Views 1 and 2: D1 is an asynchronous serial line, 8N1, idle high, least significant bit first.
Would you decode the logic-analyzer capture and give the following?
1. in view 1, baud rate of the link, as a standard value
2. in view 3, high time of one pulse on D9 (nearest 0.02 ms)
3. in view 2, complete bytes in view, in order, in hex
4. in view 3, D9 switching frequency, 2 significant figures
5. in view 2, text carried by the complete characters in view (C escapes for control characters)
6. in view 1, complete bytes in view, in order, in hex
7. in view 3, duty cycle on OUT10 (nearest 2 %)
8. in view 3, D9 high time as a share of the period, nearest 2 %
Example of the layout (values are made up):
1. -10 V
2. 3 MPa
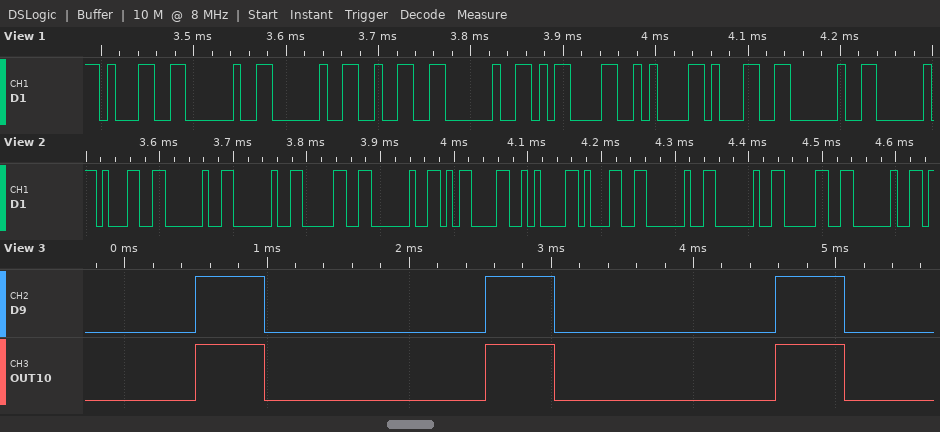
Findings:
1. 115200 baud
2. 0.48 ms
3. 31 20 20 30 20 0D 0A 31 20 20 30 20
4. 490 Hz
5. "1  0 \r\n1  0 "
6. 31 20 20 32 20 0D 0A 31 20
7. 24 %
8. 24 %
